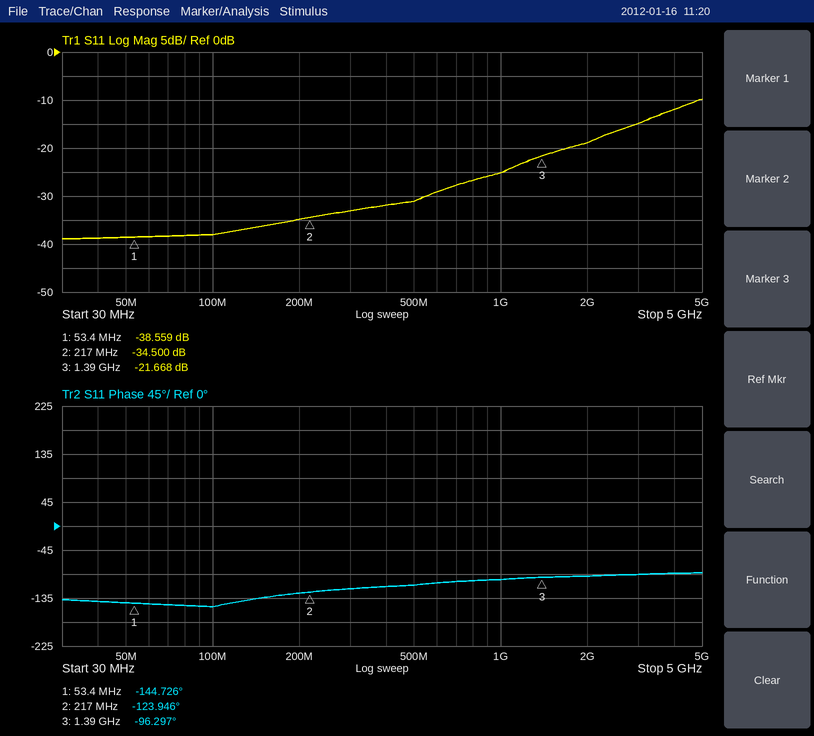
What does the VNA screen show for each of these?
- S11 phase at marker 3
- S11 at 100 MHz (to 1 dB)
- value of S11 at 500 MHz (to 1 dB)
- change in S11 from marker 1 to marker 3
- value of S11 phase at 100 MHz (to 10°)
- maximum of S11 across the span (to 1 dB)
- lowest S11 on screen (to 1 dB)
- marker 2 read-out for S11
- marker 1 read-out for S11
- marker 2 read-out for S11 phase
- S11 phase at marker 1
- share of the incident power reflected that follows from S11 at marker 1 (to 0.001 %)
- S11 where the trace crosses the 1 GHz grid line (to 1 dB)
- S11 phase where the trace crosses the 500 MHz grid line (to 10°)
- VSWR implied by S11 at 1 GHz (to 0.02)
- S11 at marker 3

-96.297°
-38 dB
-31 dB
16.891 dB
-150°
-10 dB
-39 dB
-34.500 dB
-38.559 dB
-123.946°
-144.726°
0.014 %
-25 dB
-110°
1.12
-21.668 dB
